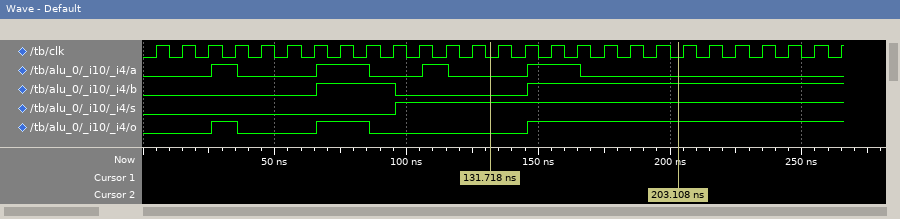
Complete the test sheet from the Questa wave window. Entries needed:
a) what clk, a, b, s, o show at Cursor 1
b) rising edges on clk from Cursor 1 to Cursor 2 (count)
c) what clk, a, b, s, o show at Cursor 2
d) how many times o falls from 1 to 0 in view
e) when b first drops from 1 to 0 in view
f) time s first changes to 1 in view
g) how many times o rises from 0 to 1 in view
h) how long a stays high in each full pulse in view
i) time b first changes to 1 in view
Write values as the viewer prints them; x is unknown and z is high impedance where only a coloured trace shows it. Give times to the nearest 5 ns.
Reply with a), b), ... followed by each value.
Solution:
a) clk=0, a=0, b=0, s=1, o=0
b) 7
c) clk=0, a=0, b=1, s=1, o=1
d) 2
e) 95 ns
f) 95 ns
g) 3
h) 10 ns, 20 ns, 10 ns, 20 ns
i) 65 ns
